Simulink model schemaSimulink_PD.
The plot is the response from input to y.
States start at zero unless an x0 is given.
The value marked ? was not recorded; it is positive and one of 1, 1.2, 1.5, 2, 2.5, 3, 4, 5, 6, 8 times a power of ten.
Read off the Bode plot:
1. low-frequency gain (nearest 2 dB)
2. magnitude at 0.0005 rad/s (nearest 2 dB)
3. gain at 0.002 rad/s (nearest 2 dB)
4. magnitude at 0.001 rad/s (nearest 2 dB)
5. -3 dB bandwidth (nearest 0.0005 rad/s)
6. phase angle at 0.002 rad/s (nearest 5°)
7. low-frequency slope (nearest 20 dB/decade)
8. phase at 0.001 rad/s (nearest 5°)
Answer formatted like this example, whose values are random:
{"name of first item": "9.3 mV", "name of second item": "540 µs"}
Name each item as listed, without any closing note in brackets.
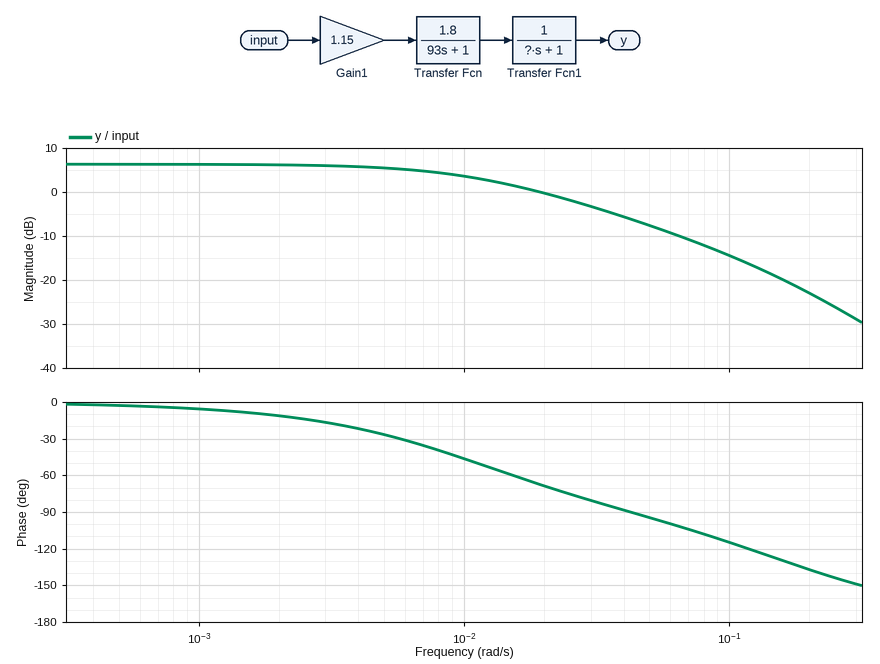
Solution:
{"low-frequency gain": "6 dB", "magnitude at 0.0005 rad/s": "6 dB", "gain at 0.002 rad/s": "6 dB", "magnitude at 0.001 rad/s": "6 dB", "-3 dB bandwidth": "0.0105 rad/s", "phase angle at 0.002 rad/s": "-10°", "low-frequency slope": "0 dB/decade", "phase at 0.001 rad/s": "-5°"}
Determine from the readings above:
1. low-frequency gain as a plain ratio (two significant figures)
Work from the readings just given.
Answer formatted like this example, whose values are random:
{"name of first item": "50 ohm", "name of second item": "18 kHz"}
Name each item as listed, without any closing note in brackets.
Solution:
{"low-frequency gain as a plain ratio": "2.0"}
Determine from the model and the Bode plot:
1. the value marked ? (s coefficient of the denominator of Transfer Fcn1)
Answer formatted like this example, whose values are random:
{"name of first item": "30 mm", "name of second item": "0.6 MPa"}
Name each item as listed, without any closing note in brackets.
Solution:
{"the value marked ?": "6"}
